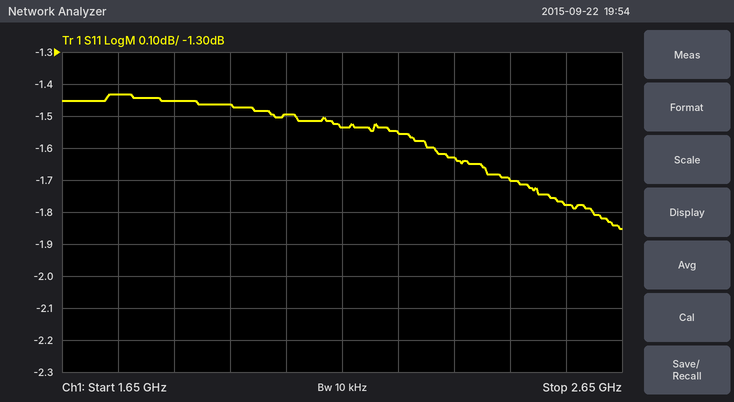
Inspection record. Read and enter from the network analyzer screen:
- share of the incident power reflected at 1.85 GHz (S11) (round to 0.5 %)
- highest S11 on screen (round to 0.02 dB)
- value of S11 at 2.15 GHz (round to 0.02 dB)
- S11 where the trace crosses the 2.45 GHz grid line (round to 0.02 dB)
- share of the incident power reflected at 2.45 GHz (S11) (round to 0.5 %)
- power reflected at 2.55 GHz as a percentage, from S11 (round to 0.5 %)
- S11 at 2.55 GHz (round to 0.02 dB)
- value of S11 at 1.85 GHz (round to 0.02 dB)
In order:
71.5 %
-1.44 dB
-1.54 dB
-1.70 dB
67.5 %
66.5 %
-1.78 dB
-1.46 dB
